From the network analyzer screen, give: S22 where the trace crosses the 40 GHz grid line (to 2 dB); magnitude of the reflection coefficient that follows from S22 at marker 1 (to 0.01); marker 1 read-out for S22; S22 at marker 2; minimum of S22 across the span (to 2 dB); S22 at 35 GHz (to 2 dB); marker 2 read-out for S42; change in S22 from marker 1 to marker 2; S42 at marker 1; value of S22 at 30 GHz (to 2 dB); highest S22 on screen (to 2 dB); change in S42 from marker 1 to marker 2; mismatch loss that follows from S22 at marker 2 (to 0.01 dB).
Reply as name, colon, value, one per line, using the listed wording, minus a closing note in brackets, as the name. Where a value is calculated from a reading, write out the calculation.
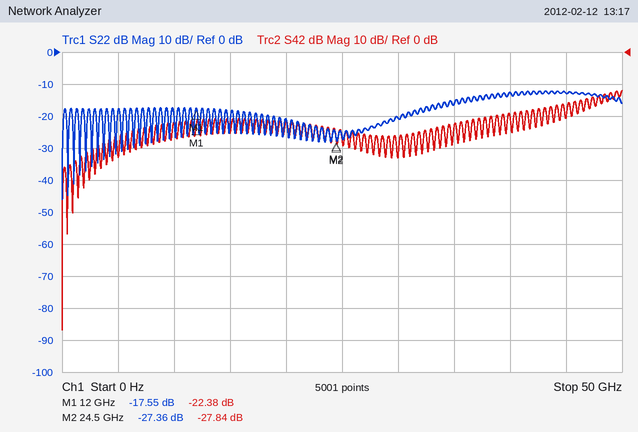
S22 where the trace crosses the 40 GHz grid line: -12 dB
magnitude of the reflection coefficient that follows from S22 at marker 1: 10^(-17.55/20) ≈ 0.13
marker 1 read-out for S22: -17.55 dB
S22 at marker 2: -27.36 dB
minimum of S22 across the span: -46 dB
S22 at 35 GHz: -16 dB
marker 2 read-out for S42: -27.84 dB
change in S22 from marker 1 to marker 2: -27.36 − (-17.55) = -9.81 dB
S42 at marker 1: -22.38 dB
value of S22 at 30 GHz: -20 dB
highest S22 on screen: -12 dB
change in S42 from marker 1 to marker 2: -27.84 − (-22.38) = -5.46 dB
mismatch loss that follows from S22 at marker 2: −10 log10(1 − 10^(-27.36/10)) ≈ 0.01 dB
